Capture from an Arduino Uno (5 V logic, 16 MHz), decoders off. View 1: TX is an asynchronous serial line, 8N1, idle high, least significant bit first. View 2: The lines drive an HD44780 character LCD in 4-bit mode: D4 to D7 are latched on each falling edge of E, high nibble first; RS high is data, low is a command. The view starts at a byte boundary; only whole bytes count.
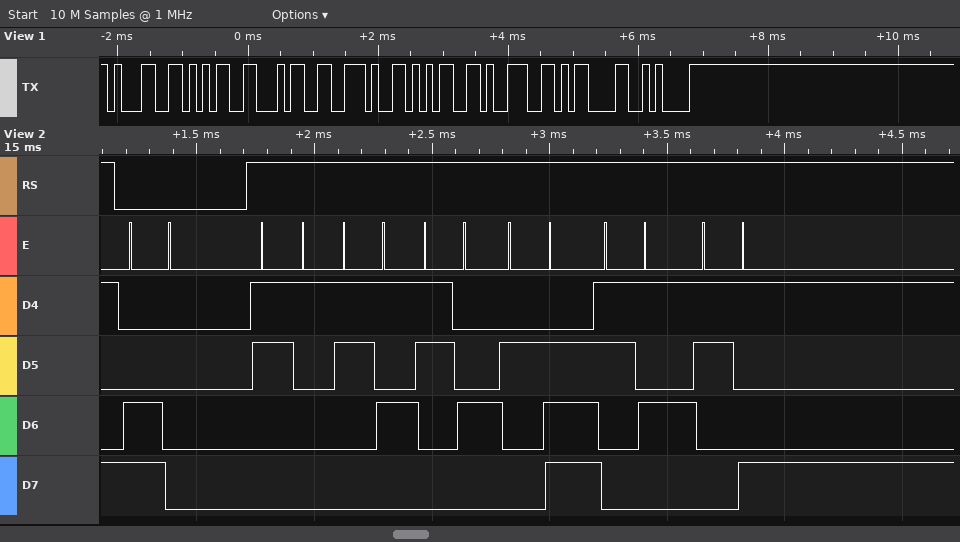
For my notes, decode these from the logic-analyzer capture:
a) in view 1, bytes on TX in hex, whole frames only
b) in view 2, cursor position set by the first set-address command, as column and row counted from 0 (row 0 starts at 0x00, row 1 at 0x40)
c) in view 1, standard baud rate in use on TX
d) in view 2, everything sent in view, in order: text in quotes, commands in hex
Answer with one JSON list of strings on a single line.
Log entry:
["31 35 34 2E 35 39 0D 0A", "column 0, row 1", "9600 baud", "0xC0 \"154.59\""]
